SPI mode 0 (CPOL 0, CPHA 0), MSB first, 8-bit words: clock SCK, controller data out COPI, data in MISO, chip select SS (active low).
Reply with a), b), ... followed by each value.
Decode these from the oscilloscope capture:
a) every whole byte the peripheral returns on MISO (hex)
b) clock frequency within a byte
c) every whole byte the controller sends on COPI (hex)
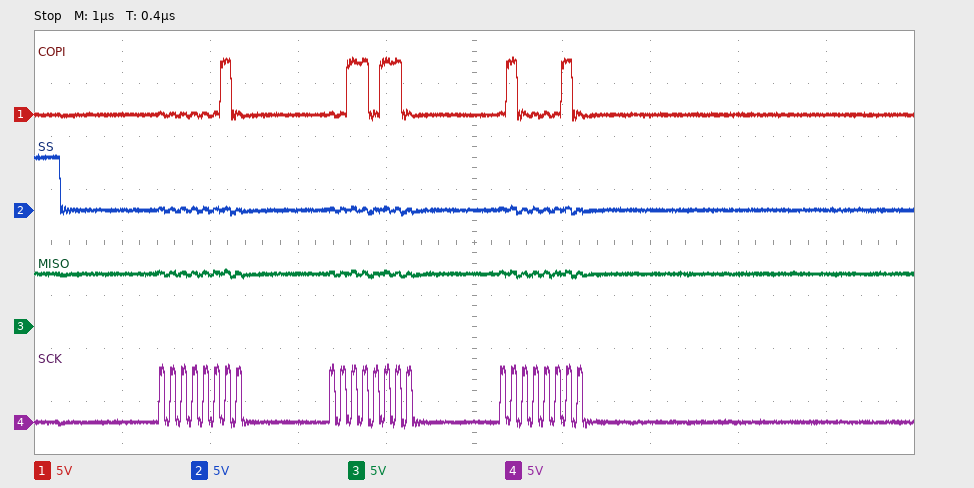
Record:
a) FF FF FF
b) 8 MHz
c) 02 36 42
